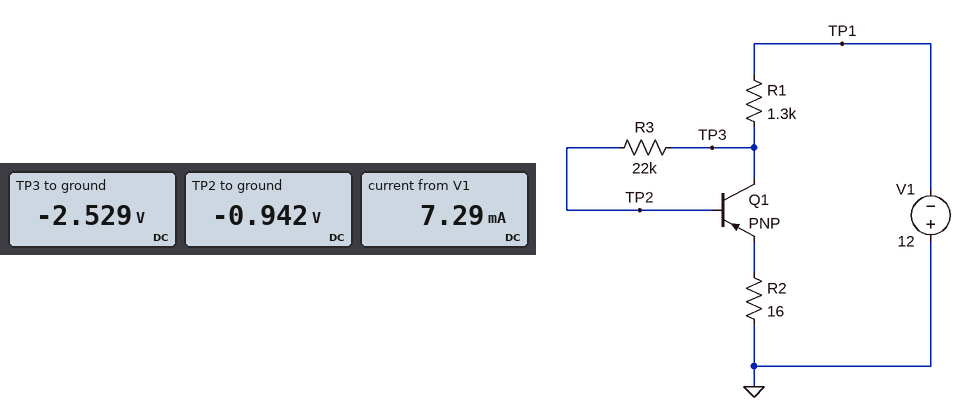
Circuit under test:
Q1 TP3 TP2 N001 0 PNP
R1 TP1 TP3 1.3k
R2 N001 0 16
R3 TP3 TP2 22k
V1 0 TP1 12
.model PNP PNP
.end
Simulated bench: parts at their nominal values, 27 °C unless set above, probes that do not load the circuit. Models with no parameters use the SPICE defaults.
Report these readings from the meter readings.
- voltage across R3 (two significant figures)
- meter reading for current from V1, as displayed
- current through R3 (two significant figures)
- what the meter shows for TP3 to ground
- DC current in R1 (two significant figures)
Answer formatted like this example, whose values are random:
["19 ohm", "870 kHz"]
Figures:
["1.6 V", "7.29 mA", "72 µA", "-2.529 V", "7.3 mA"]
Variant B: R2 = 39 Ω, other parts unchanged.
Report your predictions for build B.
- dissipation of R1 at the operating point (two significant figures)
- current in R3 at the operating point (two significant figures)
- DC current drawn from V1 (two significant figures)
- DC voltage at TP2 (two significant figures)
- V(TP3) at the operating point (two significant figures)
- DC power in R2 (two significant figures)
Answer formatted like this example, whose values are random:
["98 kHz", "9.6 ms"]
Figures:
["67 mW", "71 µA", "7.2 mA", "-1.1 V", "-2.7 V", "2.0 mW"]
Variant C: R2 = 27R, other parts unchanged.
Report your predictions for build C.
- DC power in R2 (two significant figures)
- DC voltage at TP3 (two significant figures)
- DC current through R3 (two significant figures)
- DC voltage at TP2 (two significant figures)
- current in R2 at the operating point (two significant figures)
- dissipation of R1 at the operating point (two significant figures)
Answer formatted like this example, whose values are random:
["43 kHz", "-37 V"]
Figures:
["1.4 mW", "-2.6 V", "72 µA", "-1.0 V", "7.2 mA", "68 mW"]
